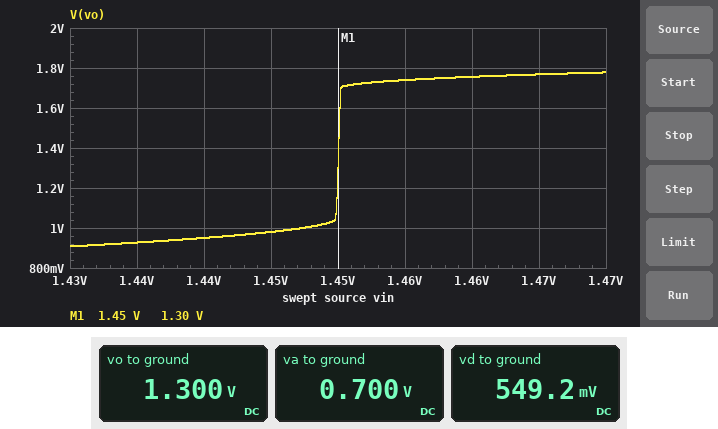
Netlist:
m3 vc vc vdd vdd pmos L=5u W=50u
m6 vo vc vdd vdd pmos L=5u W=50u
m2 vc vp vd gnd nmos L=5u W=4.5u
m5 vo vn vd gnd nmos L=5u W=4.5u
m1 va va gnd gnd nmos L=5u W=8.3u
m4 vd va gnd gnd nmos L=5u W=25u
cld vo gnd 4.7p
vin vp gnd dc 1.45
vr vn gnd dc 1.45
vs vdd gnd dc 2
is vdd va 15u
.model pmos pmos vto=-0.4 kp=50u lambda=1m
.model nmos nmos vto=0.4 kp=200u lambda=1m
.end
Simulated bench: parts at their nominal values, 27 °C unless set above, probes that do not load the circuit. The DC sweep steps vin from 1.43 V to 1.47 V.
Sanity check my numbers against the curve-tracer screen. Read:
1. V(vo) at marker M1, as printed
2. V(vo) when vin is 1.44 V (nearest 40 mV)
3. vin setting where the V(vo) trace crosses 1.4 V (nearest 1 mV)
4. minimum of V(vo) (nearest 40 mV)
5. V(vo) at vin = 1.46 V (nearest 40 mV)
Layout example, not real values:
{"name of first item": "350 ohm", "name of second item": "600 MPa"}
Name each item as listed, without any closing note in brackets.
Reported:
{"V(vo) at marker M1, as printed": "1.30 V", "V(vo) when vin is 1.44 V": "960 mV", "vin setting where the V(vo) trace crosses 1.4 V": "1.450 V", "minimum of V(vo)": "920 mV", "V(vo) at vin = 1.46 V": "1.76 V"}
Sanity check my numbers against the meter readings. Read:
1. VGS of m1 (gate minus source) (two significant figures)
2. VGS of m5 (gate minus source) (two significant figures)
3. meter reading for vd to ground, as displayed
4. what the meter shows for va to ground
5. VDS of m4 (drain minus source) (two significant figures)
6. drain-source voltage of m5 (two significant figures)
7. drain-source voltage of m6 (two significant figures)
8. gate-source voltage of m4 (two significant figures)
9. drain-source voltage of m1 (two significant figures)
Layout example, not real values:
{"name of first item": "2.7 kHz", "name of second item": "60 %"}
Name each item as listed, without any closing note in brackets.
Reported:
{"VGS of m1 (gate minus source)": "700 mV", "VGS of m5 (gate minus source)": "900 mV", "meter reading for vd to ground, as displayed": "549.2 mV", "what the meter shows for va to ground": "0.700 V", "VDS of m4 (drain minus source)": "550 mV", "drain-source voltage of m5": "750 mV", "drain-source voltage of m6": "-700 mV", "gate-source voltage of m4": "700 mV", "drain-source voltage of m1": "700 mV"}
